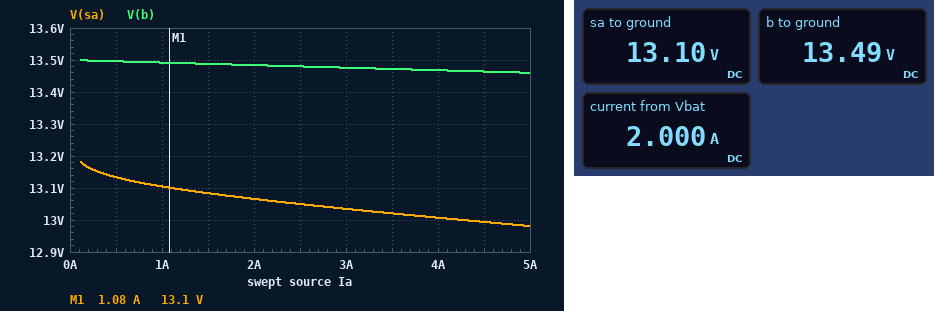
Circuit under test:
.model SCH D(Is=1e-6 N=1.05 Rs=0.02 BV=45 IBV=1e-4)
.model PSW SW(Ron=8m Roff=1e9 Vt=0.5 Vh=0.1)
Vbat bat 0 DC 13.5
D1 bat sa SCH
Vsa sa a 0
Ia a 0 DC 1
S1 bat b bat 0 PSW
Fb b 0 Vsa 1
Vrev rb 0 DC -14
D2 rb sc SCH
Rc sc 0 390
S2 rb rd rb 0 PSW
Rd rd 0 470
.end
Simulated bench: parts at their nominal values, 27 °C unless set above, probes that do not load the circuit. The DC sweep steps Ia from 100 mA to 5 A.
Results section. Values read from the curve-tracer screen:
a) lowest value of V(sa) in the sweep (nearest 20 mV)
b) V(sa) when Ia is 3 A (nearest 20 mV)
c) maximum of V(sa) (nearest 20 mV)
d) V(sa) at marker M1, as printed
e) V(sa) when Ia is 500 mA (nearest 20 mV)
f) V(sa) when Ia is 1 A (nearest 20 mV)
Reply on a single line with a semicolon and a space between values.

12.98 V; 13.04 V; 13.18 V; 13.1 V; 13.14 V; 13.10 V
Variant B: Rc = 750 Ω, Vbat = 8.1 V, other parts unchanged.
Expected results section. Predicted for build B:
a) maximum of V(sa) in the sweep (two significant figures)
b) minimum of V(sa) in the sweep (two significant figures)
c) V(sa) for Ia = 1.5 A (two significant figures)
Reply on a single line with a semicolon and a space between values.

7.8 V; 7.6 V; 7.7 V
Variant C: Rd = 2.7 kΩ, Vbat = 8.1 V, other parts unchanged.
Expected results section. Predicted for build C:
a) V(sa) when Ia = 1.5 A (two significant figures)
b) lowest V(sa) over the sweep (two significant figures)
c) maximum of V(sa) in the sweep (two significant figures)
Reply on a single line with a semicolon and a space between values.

7.7 V; 7.6 V; 7.8 V
